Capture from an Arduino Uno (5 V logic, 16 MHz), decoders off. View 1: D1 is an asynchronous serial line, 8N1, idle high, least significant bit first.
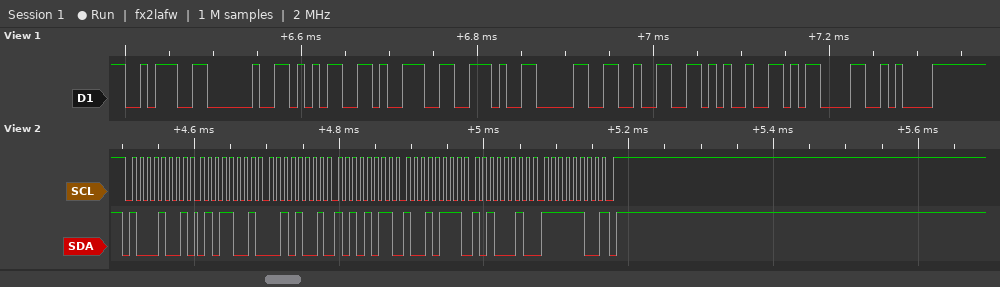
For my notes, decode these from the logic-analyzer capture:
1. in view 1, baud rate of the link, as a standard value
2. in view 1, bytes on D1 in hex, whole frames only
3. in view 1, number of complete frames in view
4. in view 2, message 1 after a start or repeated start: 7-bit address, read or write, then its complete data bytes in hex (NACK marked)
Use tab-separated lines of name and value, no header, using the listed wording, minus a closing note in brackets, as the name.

in view 1, baud rate of the link, as a standard value	115200 baud
in view 1, bytes on D1 in hex, whole frames only	3A 20 35 39 2E 30 32 25 0D 0A
in view 1, number of complete frames in view	10
in view 2, message 1 after a start or repeated start: 7-bit address, read or write, then its complete data bytes in hex	0x44 read: 59 29 AB 97 A2 FC NACK
